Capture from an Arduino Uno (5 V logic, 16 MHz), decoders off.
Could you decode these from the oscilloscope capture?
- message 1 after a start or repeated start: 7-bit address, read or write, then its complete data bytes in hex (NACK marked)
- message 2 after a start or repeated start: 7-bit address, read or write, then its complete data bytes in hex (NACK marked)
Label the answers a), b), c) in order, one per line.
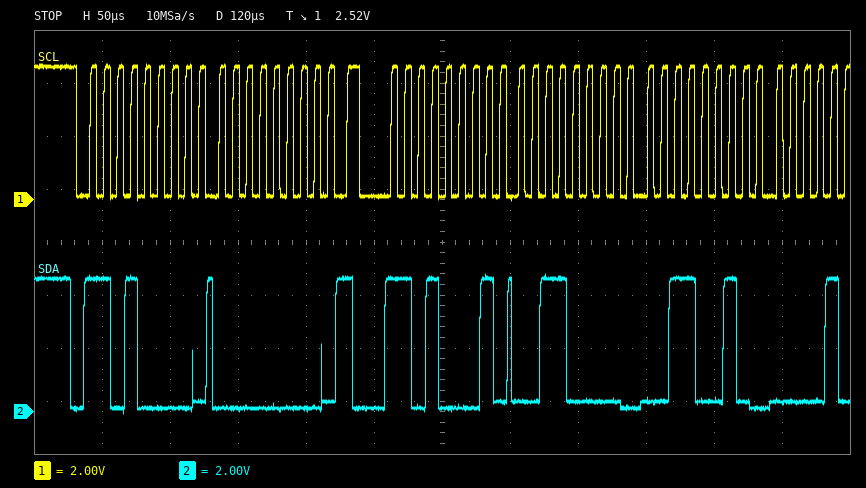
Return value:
a) 0x68 write: 00
b) 0x68 read: 30 32
